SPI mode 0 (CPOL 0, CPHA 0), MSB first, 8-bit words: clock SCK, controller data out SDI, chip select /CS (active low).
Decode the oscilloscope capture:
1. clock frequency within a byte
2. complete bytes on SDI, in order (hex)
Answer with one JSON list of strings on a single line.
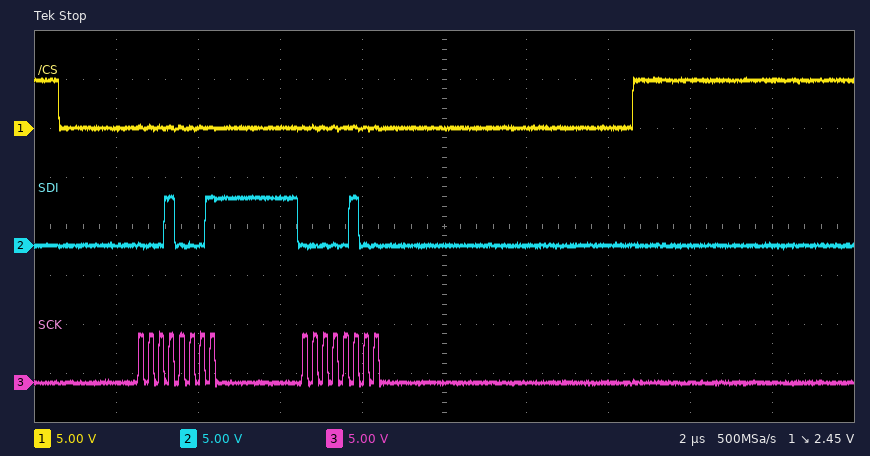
["4 MHz", "0x11 0x04"]
